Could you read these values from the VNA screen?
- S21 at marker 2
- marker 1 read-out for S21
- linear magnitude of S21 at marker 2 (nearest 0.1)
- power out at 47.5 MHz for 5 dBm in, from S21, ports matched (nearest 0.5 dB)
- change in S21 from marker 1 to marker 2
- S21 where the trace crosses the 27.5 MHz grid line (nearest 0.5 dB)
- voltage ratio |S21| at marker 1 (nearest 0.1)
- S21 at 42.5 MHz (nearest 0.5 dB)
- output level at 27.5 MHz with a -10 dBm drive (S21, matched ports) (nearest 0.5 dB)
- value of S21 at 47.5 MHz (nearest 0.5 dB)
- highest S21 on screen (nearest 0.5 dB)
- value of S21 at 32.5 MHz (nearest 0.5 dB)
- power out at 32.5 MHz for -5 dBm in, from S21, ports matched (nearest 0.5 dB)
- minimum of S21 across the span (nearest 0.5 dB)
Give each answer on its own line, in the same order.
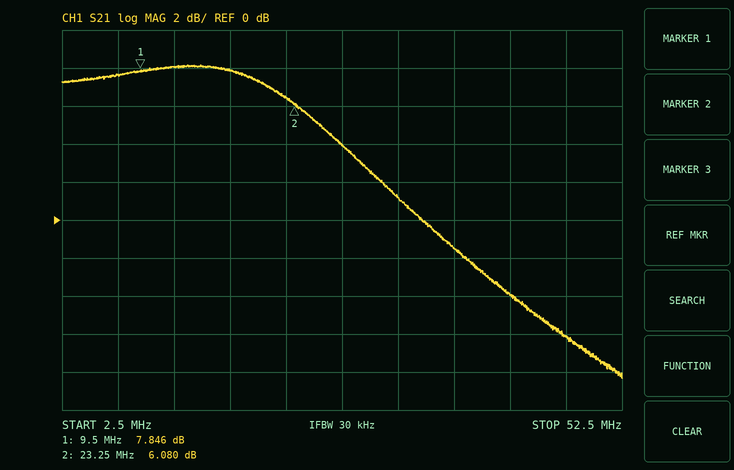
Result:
6.080 dB
7.846 dB
2.0
-1.0 dBm
-1.766 dB
4.0 dB
2.5
-4.0 dB
-6.0 dBm
-6.0 dB
8.0 dB
1.0 dB
-4.0 dBm
-8.5 dB
